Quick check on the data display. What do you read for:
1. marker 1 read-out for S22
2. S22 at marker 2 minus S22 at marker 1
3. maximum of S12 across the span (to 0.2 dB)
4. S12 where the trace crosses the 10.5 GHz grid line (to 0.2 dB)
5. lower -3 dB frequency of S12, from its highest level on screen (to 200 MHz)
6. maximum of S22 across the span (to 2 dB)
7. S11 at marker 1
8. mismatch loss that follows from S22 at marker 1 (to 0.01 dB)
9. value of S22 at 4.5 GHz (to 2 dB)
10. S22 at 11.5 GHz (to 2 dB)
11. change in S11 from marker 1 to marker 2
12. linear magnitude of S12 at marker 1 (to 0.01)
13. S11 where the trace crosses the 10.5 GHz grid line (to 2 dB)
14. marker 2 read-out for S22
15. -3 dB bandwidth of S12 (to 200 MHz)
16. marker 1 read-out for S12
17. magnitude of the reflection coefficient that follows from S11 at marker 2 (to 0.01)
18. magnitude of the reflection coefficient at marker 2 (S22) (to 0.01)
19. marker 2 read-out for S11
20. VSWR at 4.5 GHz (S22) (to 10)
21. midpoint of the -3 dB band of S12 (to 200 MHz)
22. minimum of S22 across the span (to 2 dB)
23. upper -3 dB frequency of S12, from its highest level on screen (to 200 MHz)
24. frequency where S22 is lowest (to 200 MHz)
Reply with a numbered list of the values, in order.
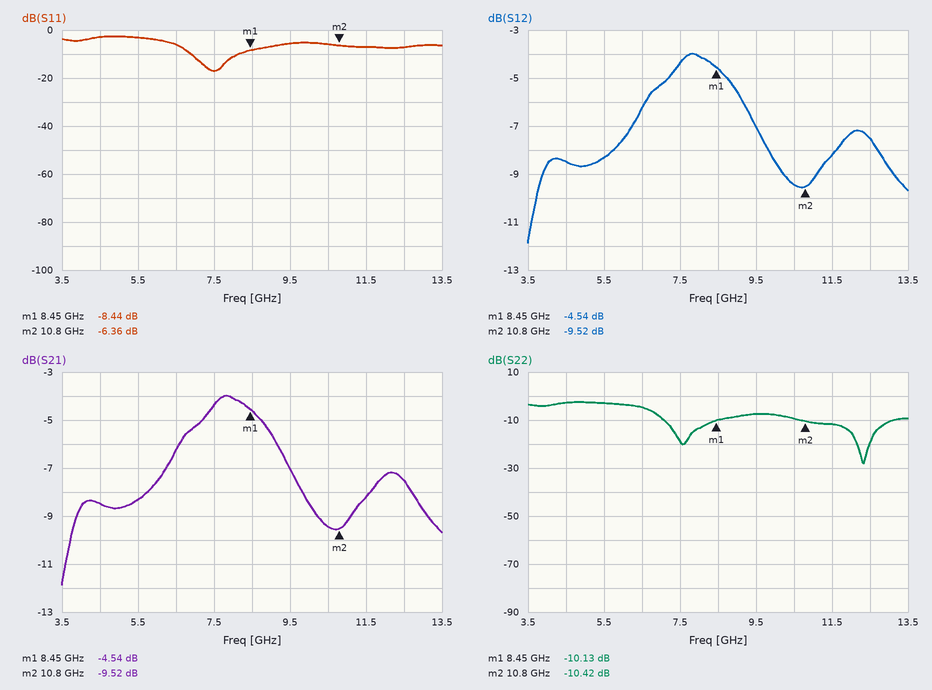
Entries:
1. -10.13 dB
2. -0.29 dB
3. -4.0 dB
4. -9.4 dB
5. 6.2 GHz
6. -2 dB
7. -8.44 dB
8. 0.44 dB
9. -2 dB
10. -12 dB
11. 2.08 dB
12. 0.59
13. -6 dB
14. -10.42 dB
15. 3.2 GHz
16. -4.54 dB
17. 0.48
18. 0.30
19. -6.36 dB
20. 10
21. 7.8 GHz
22. -28 dB
23. 9.4 GHz
24. 12.4 GHz
